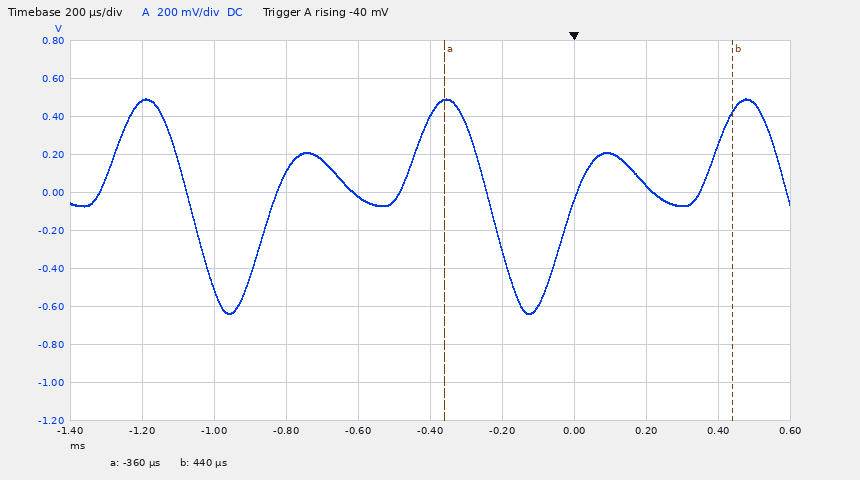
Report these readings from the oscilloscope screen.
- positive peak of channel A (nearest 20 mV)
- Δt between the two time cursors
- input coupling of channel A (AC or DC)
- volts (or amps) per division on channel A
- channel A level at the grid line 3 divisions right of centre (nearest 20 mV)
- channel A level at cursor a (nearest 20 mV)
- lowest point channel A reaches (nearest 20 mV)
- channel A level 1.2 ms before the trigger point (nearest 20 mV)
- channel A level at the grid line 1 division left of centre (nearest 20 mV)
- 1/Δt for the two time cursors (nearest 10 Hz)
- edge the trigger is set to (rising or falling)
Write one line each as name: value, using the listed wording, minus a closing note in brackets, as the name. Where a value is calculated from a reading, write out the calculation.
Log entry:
positive peak of channel A: 500 mV
Δt between the two time cursors: 440 µs − (-360 µs) = 800 µs
input coupling of channel A: DC
volts (or amps) per division on channel A: 200 mV
channel A level at the grid line 3 divisions right of centre: 40 mV
channel A level at cursor a: 480 mV
lowest point channel A reaches: -640 mV
channel A level 1.2 ms before the trigger point: 480 mV
channel A level at the grid line 1 division left of centre: -20 mV
1/Δt for the two time cursors: 1 / 800 µs ≈ 1.25 kHz
edge the trigger is set to: rising
